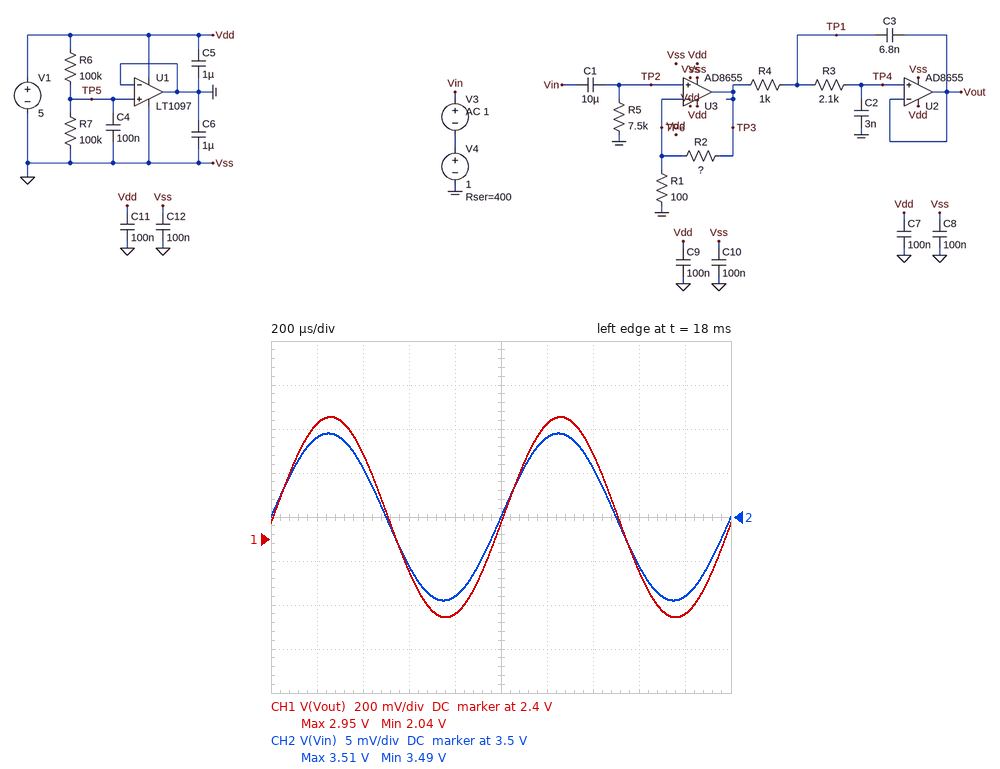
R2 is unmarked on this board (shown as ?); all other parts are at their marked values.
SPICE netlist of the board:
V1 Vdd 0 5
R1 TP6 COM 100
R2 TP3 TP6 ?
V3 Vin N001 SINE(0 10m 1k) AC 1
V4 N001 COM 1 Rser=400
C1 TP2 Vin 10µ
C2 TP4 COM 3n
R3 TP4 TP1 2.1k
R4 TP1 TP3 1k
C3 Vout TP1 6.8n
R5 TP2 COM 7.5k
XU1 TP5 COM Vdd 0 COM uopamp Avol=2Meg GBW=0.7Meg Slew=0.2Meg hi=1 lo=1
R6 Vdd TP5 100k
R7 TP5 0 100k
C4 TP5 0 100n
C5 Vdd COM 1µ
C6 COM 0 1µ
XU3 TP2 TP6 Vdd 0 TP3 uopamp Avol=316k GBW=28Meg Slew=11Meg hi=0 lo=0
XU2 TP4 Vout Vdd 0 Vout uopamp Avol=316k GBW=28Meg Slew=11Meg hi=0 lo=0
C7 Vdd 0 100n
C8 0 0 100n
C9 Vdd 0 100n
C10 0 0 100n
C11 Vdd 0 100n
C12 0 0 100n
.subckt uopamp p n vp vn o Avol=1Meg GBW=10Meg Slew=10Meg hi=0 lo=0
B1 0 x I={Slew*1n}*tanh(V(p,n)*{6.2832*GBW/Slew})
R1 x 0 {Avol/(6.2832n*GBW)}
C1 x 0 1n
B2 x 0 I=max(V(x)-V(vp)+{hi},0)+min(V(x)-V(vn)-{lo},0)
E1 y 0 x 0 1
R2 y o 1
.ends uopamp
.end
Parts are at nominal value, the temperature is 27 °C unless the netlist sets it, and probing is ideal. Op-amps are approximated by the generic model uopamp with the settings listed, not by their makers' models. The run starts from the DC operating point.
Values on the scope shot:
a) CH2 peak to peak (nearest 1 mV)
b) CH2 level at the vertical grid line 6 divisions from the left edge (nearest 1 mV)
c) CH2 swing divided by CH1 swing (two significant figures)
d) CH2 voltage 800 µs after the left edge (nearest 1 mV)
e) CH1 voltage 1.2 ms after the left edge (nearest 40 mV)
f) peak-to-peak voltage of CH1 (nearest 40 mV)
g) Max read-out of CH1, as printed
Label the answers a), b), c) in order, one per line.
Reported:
a) 19 mV
b) 3.509 V
c) 0.021
d) 3.491 V
e) 2.92 V
f) 920 mV
g) 2.95 V
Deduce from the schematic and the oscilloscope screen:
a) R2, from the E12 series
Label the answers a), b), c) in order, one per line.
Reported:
a) 4.7 kΩ
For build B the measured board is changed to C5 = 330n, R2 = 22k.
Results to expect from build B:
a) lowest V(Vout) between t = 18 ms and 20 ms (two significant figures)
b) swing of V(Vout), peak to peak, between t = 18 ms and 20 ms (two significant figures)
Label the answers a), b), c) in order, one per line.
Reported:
a) 400 mV
b) 4.2 V
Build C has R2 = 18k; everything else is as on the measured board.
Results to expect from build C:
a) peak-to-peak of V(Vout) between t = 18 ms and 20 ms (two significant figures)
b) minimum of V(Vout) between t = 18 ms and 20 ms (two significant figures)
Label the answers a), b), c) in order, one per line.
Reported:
a) 3.4 V
b) 780 mV
